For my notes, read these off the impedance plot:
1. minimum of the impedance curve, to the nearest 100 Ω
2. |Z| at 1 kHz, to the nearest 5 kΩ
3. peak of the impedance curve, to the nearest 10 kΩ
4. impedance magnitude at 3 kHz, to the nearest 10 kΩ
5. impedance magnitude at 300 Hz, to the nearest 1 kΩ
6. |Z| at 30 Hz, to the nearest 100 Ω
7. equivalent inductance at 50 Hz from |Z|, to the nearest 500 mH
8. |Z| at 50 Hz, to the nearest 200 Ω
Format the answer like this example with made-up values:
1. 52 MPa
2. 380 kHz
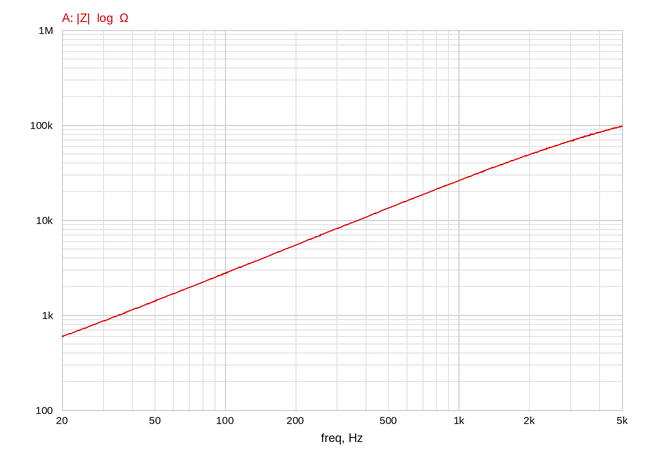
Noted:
1. 600 Ω
2. 25 kΩ
3. 100 kΩ
4. 70 kΩ
5. 8 kΩ
6. 900 Ω
7. 4.5 H
8. 1.4 kΩ
